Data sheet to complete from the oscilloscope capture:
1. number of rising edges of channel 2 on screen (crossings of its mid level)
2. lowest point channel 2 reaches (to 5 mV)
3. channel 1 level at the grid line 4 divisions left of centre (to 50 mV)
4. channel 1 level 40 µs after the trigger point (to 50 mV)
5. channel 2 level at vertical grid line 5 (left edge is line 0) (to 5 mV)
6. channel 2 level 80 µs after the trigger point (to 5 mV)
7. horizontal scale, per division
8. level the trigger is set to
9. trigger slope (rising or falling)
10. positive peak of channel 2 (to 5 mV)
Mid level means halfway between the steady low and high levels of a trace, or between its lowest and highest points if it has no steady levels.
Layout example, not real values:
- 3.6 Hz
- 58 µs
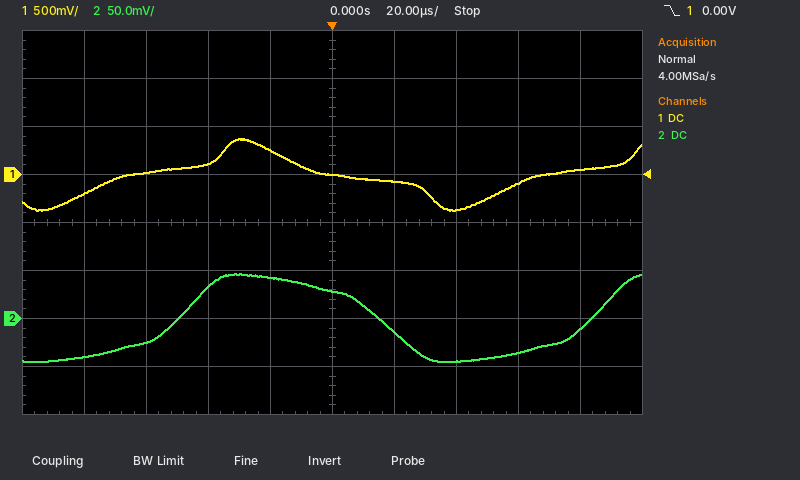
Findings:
- 2
- -45 mV
- -200 mV
- -350 mV
- 30 mV
- -10 mV
- 20 µs
- 0.00 V
- falling
- 45 mV
